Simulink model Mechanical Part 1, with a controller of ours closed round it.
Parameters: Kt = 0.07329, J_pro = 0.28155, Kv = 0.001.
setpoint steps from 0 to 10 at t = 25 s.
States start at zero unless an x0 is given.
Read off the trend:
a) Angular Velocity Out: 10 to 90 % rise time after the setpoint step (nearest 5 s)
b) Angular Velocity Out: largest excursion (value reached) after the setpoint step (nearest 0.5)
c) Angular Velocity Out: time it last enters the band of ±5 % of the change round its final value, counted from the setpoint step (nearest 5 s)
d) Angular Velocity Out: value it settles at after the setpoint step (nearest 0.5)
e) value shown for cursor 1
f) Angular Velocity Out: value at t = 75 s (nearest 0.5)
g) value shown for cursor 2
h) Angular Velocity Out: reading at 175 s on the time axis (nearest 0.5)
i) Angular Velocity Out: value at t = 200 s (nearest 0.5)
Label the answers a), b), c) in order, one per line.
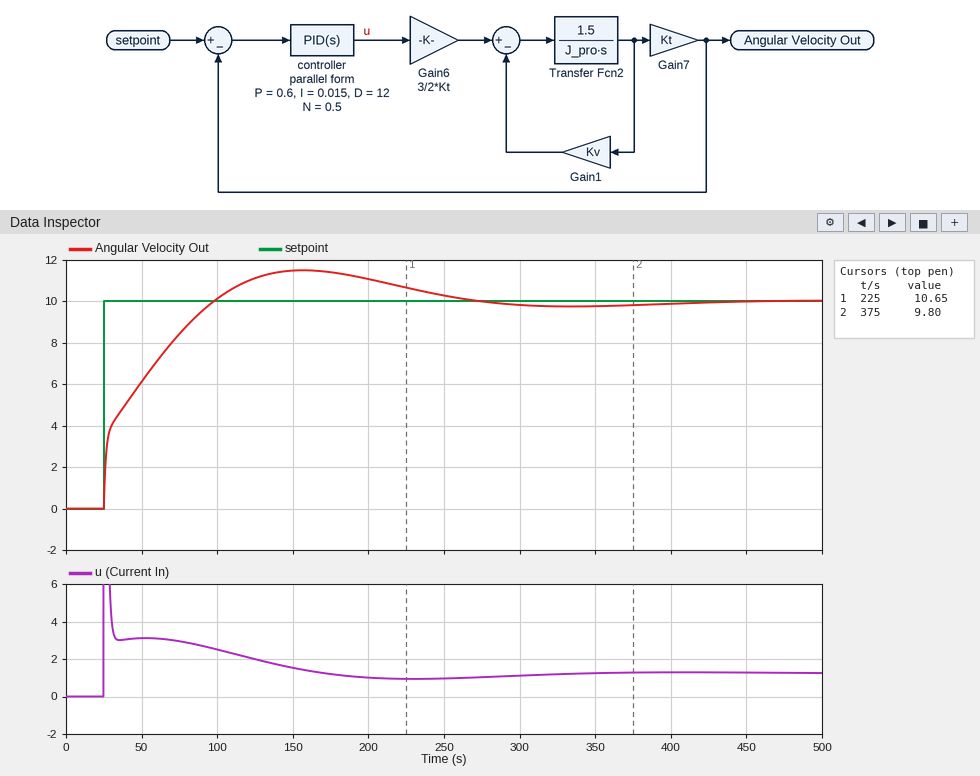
a) 55 s
b) 11.5
c) 210 s
d) 10.0
e) 10.65
f) 8.5
g) 9.80
h) 11.5
i) 11.0
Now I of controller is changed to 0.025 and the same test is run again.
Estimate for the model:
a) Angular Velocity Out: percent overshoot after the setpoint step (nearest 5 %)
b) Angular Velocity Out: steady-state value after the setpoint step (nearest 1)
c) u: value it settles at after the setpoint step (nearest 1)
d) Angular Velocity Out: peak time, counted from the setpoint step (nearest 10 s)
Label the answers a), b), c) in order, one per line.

a) 20 %
b) 10
c) 1
d) 100 s
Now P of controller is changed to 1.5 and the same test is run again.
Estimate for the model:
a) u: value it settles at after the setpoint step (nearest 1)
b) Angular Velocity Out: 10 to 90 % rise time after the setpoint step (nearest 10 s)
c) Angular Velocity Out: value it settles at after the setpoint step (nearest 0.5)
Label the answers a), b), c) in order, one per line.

a) 1
b) 40 s
c) 10.0
